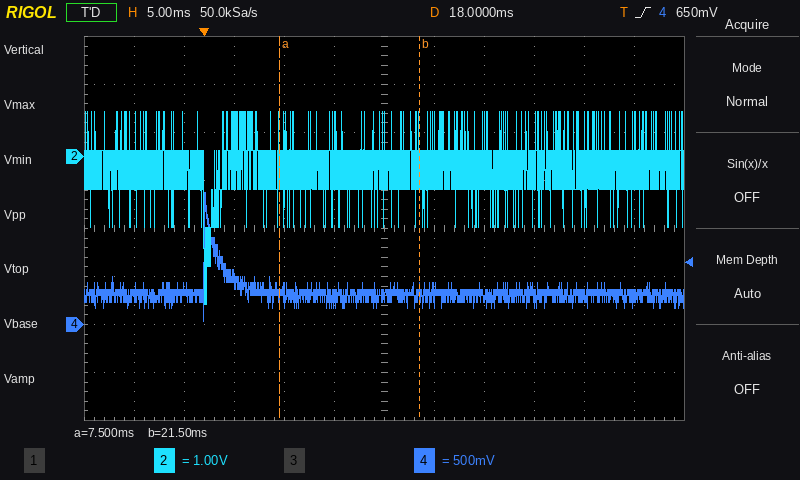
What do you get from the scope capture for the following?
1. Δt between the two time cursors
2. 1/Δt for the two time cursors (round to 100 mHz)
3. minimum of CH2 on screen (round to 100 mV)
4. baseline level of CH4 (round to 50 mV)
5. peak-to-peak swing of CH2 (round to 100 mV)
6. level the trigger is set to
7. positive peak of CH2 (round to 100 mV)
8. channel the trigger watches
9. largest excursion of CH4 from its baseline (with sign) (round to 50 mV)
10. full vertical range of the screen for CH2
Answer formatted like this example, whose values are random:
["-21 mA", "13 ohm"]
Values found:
["14.0 ms", "71.4 Hz", "-3.1 V", "300 mV", "4.0 V", "650 mV", "900 mV", "CH4", "+1.10 V", "8 V"]
